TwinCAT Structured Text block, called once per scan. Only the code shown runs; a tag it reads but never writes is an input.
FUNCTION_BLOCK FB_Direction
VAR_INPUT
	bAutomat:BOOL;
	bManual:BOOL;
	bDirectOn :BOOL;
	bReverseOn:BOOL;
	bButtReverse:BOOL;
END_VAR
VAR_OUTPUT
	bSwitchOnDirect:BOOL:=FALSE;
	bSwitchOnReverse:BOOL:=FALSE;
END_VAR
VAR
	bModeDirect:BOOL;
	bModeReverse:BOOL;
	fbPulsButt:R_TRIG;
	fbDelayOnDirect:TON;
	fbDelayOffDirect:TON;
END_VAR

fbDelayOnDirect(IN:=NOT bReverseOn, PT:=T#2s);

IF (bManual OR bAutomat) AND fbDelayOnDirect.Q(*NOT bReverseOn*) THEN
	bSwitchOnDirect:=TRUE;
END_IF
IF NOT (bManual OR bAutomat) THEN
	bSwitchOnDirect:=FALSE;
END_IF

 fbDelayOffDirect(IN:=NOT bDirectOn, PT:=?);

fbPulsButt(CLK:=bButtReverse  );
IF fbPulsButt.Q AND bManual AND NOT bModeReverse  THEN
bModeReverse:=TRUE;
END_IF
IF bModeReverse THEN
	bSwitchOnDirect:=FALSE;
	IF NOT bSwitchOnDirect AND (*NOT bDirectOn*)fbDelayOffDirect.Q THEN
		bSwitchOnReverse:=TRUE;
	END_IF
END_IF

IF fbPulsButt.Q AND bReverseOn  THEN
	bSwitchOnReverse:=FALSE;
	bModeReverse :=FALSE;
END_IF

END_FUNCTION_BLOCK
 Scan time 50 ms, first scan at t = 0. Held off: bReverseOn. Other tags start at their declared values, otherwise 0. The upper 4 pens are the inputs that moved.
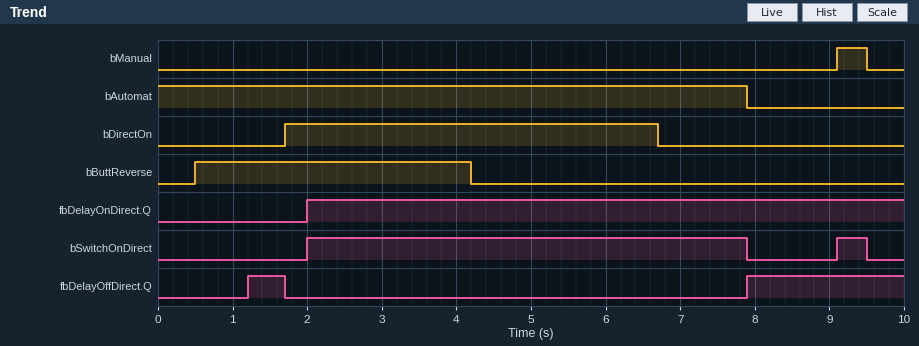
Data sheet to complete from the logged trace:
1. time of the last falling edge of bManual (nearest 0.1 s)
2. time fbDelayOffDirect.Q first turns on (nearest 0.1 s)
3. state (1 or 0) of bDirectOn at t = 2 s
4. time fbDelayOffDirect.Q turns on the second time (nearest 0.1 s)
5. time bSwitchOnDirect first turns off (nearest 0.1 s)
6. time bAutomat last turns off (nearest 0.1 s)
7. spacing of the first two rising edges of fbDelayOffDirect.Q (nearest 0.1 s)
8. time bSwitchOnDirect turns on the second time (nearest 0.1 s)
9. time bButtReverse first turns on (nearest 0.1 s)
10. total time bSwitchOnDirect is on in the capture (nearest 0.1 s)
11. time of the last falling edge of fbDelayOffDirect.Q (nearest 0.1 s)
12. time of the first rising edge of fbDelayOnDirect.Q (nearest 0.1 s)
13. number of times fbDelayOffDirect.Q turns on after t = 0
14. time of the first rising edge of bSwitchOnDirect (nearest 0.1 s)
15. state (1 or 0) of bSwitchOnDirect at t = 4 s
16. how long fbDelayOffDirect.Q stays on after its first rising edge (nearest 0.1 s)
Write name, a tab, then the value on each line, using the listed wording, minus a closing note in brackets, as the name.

time of the last falling edge of bManual	9.5 s
time fbDelayOffDirect.Q first turns on	1.2 s
state (1 or 0) of bDirectOn at t = 2 s	1
time fbDelayOffDirect.Q turns on the second time	7.9 s
time bSwitchOnDirect first turns off	7.9 s
time bAutomat last turns off	7.9 s
spacing of the first two rising edges of fbDelayOffDirect.Q	6.7 s
time bSwitchOnDirect turns on the second time	9.1 s
time bButtReverse first turns on	0.5 s
total time bSwitchOnDirect is on in the capture	6.3 s
time of the last falling edge of fbDelayOffDirect.Q	1.7 s
time of the first rising edge of fbDelayOnDirect.Q	2.0 s
number of times fbDelayOffDirect.Q turns on after t = 0	2
time of the first rising edge of bSwitchOnDirect	2.0 s
state (1 or 0) of bSwitchOnDirect at t = 4 s	1
how long fbDelayOffDirect.Q stays on after its first rising edge	0.5 s
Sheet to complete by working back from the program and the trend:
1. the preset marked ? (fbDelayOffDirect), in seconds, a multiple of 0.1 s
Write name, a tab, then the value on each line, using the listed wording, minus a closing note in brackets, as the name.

the preset marked ? (fbDelayOffDirect), in seconds, a multiple of 0.1 s	1.2 s
